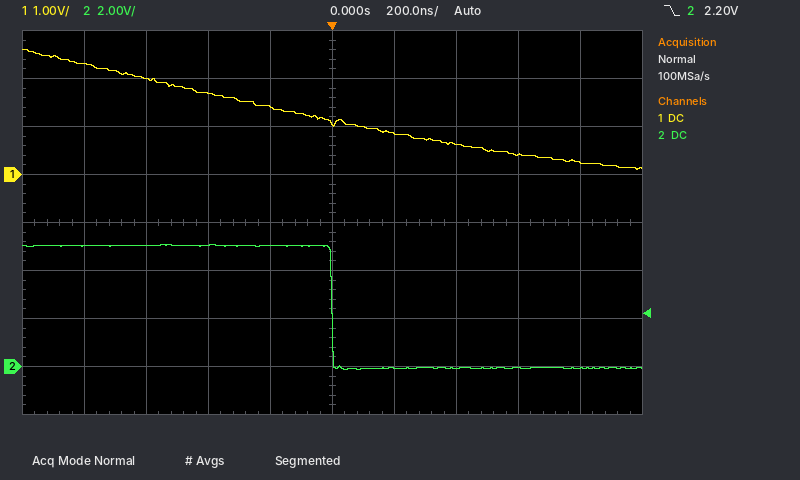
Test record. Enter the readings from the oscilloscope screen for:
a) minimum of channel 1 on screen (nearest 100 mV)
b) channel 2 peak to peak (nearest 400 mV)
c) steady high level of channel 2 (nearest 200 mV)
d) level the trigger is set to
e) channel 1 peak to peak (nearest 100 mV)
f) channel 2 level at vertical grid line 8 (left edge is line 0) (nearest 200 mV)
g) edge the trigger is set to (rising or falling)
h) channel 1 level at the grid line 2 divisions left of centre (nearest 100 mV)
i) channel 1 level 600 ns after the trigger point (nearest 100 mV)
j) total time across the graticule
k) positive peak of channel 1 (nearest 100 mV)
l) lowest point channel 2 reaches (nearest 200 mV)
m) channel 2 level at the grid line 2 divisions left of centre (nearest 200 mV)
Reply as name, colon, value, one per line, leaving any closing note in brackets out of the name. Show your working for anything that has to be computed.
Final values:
minimum of channel 1 on screen: 100 mV
channel 2 peak to peak: 5.2 V
steady high level of channel 2: 5.0 V
level the trigger is set to: 2.20 V
channel 1 peak to peak: 2.6 V − (100 mV) = 2.5 V
channel 2 level at vertical grid line 8 (left edge is line 0): 0.0 V
edge the trigger is set to: falling
channel 1 level at the grid line 2 divisions left of centre: 1.7 V
channel 1 level 600 ns after the trigger point: 400 mV
total time across the graticule: 2 µs
positive peak of channel 1: 2.6 V
lowest point channel 2 reaches: -200 mV
channel 2 level at the grid line 2 divisions left of centre: 5.0 V
